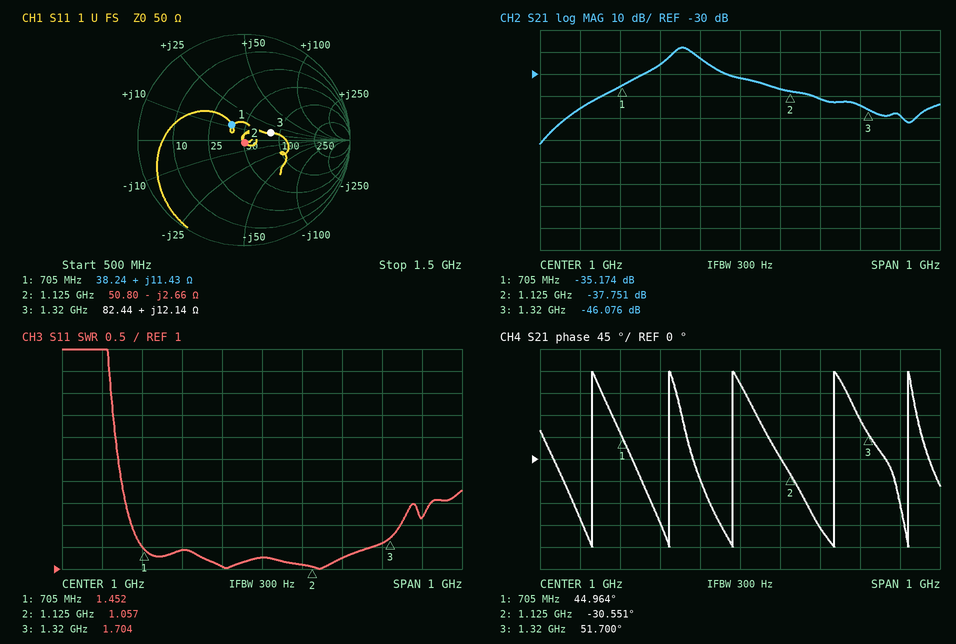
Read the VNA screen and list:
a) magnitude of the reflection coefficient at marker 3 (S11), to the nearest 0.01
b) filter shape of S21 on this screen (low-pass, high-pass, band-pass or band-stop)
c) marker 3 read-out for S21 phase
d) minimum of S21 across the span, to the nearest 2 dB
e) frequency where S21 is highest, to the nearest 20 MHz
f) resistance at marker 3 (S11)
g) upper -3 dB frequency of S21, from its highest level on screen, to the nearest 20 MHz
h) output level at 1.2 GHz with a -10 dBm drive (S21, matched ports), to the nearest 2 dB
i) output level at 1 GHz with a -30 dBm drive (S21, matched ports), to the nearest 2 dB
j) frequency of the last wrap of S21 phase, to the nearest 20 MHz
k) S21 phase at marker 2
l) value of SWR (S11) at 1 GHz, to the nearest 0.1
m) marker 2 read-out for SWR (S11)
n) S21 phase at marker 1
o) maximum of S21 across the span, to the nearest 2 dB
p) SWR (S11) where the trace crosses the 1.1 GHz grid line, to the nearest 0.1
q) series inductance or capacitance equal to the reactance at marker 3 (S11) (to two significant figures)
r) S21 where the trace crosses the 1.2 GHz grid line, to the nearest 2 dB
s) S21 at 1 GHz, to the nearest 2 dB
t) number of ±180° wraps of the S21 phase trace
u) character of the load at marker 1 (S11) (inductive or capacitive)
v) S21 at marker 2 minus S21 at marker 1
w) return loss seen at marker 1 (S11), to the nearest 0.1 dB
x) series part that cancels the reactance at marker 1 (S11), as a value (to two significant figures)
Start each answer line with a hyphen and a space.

- 0.26
- band-pass
- 51.700°
- -62 dB
- 860 MHz
- 82.44 Ω
- 880 MHz
- -52 dBm
- -62 dBm
- 1.42 GHz
- -30.551°
- 1.3
- 1.057
- 44.964°
- -18 dB
- 1.1
- 1.5 nH
- -42 dB
- -32 dB
- 5
- inductive
- -2.577 dB
- 14.7 dB
- 20 pF
